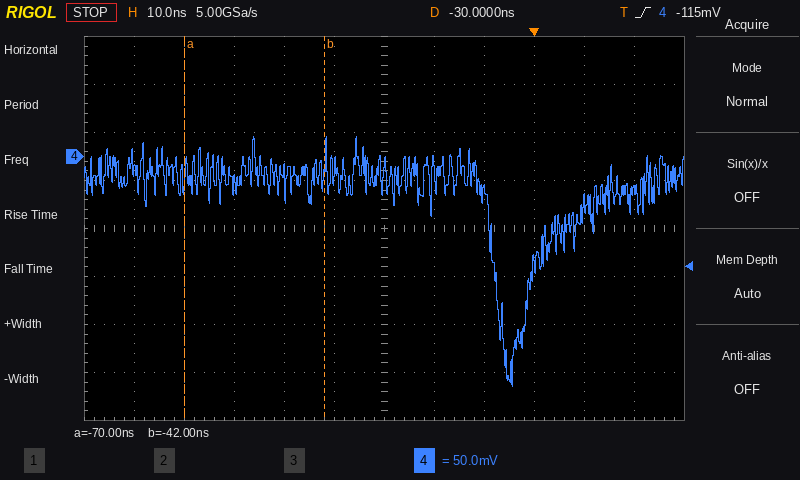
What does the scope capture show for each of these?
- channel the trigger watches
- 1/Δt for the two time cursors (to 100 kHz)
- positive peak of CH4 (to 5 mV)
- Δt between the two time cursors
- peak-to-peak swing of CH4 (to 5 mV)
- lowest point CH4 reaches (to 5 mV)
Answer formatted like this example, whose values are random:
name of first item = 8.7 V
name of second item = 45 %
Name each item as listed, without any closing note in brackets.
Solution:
channel the trigger watches = CH4
1/Δt for the two time cursors = 35.7 MHz
positive peak of CH4 = 20 mV
Δt between the two time cursors = 28 ns
peak-to-peak swing of CH4 = 260 mV
lowest point CH4 reaches = -240 mV
